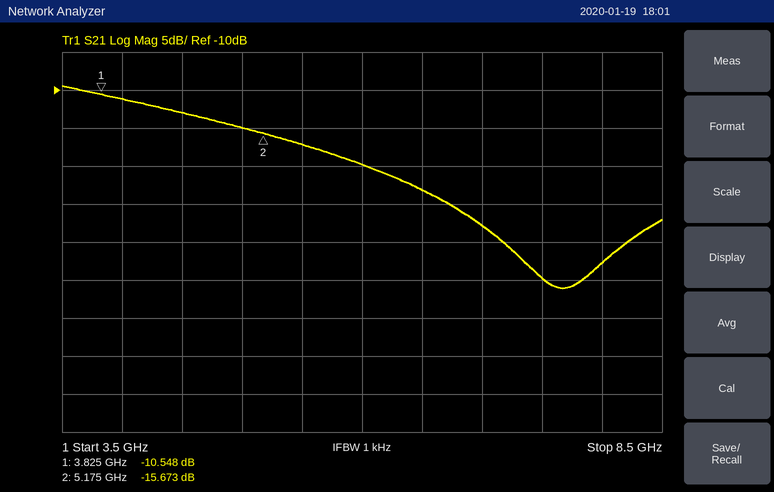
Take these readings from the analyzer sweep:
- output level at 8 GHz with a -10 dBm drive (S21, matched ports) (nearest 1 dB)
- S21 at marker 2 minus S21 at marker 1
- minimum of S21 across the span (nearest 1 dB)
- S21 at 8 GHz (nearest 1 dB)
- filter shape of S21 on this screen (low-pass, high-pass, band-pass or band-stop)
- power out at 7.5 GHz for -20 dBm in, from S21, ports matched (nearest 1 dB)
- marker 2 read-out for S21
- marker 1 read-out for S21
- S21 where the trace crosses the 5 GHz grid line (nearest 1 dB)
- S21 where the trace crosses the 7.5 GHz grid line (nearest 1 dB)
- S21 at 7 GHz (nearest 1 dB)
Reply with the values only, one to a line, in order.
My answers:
-43 dBm
-5.125 dB
-36 dB
-33 dB
low-pass
-55 dBm
-15.673 dB
-10.548 dB
-15 dB
-35 dB
-28 dB
